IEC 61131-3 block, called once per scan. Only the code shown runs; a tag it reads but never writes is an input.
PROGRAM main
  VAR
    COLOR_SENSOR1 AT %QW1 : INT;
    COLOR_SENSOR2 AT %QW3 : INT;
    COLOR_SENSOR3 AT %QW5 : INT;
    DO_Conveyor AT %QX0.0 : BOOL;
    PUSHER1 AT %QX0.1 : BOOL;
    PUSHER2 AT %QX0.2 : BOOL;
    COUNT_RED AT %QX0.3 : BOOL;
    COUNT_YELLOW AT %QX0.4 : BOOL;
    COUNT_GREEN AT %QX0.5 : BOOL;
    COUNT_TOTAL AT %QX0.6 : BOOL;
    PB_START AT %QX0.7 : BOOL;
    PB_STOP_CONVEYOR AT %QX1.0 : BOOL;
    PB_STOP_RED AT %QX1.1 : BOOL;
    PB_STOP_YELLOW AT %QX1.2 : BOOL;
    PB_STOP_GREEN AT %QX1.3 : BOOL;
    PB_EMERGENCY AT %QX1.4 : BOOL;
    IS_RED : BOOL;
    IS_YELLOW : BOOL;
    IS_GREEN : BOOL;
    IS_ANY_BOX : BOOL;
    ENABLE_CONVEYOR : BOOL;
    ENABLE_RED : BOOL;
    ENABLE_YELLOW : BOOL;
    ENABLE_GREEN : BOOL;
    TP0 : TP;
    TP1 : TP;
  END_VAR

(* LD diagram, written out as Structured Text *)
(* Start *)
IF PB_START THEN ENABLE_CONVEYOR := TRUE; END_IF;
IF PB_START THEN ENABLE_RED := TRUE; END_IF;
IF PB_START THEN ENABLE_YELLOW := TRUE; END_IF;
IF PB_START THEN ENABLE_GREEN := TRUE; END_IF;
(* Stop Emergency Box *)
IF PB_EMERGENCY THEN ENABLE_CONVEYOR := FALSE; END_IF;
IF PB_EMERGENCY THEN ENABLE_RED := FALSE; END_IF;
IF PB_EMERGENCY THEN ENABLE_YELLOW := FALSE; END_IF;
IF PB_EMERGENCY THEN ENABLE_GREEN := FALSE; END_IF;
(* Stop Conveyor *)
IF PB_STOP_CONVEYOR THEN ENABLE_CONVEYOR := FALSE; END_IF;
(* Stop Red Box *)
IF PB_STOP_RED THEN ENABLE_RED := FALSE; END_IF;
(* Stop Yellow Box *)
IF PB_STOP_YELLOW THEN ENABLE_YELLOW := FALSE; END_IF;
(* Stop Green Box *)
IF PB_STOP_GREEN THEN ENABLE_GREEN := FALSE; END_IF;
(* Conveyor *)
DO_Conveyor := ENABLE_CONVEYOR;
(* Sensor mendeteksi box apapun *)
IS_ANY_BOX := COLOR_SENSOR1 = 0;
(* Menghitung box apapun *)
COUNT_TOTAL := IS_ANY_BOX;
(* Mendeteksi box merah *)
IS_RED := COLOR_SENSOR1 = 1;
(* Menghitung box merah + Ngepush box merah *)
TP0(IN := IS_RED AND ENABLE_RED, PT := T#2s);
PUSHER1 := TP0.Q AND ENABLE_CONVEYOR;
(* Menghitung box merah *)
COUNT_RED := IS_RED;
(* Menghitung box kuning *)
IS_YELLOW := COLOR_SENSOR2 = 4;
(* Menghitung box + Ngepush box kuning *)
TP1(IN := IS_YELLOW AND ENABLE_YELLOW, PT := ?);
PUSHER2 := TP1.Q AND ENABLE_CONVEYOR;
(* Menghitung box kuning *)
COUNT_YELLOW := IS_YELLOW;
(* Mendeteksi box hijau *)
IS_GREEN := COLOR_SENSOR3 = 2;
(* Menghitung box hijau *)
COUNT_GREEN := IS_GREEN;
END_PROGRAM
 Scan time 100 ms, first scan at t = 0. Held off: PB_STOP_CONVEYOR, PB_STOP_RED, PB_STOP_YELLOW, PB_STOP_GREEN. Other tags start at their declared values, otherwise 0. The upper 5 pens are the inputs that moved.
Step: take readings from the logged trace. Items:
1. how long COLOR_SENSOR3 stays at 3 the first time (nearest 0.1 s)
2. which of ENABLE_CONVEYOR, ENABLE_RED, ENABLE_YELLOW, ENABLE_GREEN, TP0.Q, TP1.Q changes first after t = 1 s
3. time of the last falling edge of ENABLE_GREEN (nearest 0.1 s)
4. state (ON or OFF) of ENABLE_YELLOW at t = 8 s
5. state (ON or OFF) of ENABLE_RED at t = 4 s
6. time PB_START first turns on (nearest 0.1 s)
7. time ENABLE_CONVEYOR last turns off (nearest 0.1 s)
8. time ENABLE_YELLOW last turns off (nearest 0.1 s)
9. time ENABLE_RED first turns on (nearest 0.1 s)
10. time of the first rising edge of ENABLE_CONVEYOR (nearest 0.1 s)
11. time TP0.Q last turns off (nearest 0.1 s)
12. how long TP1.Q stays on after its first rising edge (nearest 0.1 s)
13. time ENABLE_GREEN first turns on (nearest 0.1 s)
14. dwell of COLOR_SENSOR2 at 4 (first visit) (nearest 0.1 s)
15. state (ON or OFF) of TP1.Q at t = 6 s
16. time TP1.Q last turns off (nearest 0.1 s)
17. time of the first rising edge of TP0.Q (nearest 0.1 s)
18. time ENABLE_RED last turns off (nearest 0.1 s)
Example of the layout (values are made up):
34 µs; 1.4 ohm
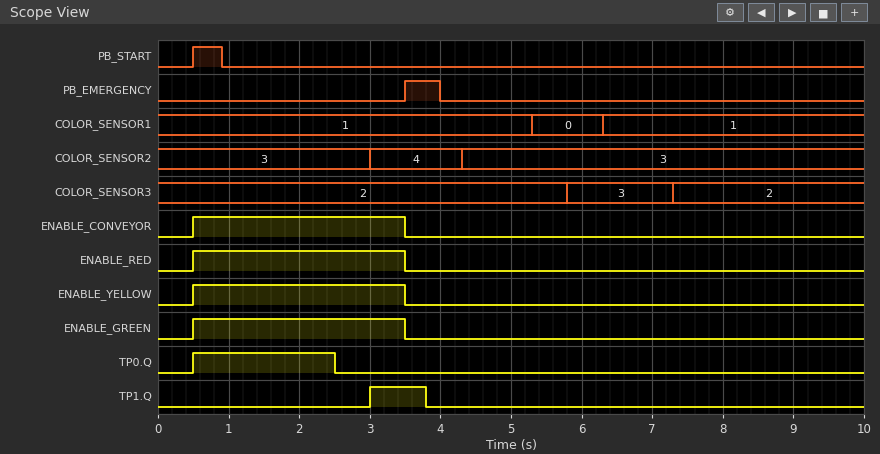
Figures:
1.5 s; TP0.Q; 3.5 s; OFF; OFF; 0.5 s; 3.5 s; 3.5 s; 0.5 s; 0.5 s; 2.5 s; 0.8 s; 0.5 s; 1.3 s; OFF; 3.8 s; 0.5 s; 3.5 s
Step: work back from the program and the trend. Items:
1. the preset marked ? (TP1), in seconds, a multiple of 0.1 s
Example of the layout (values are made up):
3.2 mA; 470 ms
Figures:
0.8 s
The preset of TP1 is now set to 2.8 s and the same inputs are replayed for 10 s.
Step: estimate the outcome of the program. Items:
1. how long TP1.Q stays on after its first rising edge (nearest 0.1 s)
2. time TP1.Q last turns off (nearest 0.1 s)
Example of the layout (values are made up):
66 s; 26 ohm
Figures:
2.8 s; 5.8 s
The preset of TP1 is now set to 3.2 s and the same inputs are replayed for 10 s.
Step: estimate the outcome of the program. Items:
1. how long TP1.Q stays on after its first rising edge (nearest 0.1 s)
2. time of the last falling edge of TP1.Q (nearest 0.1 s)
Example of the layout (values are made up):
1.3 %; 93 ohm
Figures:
3.2 s; 6.2 s
